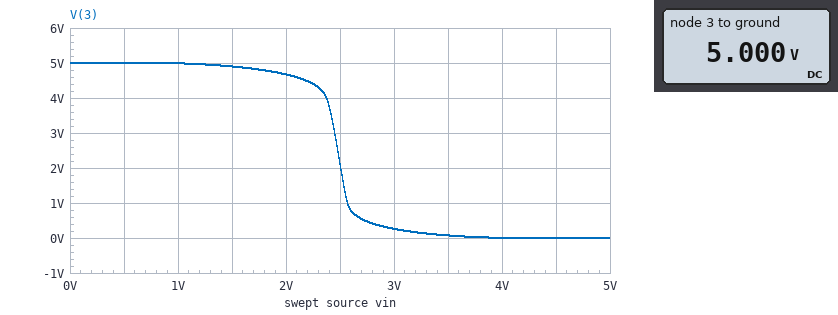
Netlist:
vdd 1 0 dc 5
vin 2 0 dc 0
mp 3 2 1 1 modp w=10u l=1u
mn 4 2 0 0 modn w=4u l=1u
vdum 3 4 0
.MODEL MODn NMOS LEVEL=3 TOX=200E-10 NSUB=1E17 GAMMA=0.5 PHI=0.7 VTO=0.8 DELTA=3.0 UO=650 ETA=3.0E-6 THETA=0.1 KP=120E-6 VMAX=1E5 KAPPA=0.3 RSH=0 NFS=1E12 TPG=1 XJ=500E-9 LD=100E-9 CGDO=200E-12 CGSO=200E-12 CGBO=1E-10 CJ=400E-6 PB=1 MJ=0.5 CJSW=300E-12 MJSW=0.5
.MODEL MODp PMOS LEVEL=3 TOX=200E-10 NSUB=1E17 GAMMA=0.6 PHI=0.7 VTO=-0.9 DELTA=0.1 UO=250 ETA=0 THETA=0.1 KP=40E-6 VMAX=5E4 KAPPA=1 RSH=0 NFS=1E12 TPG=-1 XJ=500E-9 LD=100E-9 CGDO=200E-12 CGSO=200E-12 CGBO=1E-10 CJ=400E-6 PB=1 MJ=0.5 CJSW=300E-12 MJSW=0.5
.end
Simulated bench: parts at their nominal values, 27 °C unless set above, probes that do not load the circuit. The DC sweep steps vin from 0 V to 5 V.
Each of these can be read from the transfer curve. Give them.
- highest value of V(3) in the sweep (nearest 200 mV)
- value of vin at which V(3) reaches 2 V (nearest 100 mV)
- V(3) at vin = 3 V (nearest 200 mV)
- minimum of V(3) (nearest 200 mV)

5.0 V
2.5 V
200 mV
0 V
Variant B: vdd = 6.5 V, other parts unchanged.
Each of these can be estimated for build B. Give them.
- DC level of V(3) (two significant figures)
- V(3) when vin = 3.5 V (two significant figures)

6.5 V
930 mV
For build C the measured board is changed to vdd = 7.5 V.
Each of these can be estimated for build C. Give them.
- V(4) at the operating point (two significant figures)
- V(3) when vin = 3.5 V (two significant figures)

7.5 V
6.2 V
